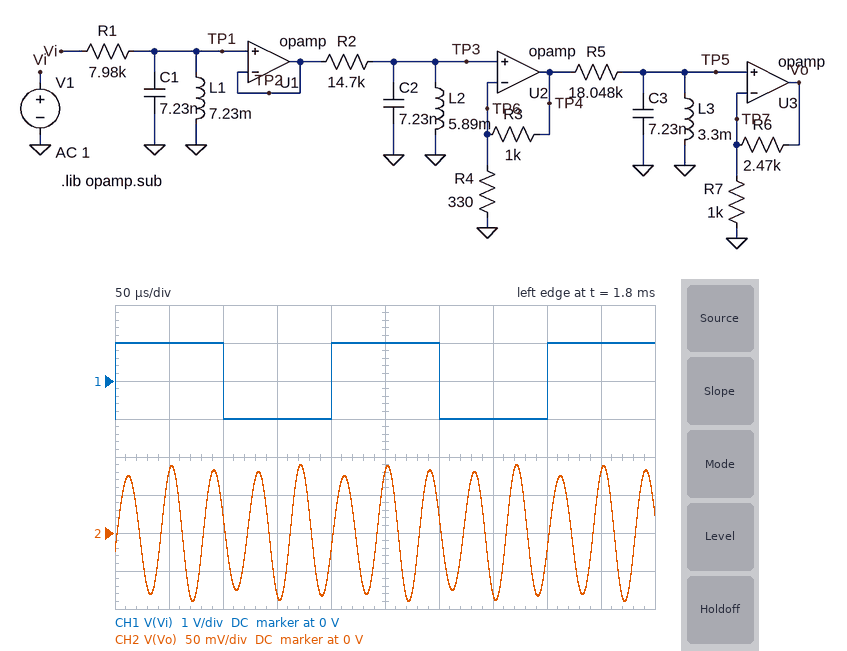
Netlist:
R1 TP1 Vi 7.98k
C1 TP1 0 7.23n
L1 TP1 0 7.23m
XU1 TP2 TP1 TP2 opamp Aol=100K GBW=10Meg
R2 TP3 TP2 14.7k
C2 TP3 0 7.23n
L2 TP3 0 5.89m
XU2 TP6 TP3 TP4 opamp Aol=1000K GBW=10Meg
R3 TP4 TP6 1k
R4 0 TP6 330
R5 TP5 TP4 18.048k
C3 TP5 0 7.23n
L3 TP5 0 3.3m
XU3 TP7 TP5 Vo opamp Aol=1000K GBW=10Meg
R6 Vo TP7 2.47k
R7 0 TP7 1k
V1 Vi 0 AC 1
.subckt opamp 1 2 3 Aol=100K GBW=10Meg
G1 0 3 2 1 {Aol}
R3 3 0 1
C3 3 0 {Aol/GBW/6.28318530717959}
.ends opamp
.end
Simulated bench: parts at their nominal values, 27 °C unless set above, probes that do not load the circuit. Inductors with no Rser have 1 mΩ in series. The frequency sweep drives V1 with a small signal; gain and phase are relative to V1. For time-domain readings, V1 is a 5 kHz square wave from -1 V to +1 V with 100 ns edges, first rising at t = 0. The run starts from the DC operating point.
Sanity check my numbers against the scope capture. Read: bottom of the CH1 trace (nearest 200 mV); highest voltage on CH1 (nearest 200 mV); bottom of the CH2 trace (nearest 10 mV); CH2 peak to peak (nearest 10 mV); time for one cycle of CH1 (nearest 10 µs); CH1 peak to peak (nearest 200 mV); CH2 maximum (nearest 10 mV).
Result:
-1.0 V
1.0 V
-90 mV
180 mV
200 µs
2.0 V
90 mV
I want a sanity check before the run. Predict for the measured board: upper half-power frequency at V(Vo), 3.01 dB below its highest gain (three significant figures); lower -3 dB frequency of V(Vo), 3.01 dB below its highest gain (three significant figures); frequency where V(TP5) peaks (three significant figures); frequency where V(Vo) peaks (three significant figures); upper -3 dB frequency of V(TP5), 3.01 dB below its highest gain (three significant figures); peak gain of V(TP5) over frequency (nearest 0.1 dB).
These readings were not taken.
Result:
25.0 kHz
23.4 kHz
24.3 kHz
24.3 kHz
25.0 kHz
-17.4 dB
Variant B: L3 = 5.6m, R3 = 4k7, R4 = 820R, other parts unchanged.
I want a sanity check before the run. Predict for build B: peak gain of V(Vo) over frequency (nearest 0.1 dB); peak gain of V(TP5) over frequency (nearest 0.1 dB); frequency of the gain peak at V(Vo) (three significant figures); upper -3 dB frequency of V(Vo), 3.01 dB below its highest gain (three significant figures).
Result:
19.2 dB
8.4 dB
24.7 kHz
25.2 kHz
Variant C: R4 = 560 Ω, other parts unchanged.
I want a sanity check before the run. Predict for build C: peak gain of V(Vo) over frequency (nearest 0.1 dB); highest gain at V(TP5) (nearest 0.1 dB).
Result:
-9.8 dB
-20.6 dB
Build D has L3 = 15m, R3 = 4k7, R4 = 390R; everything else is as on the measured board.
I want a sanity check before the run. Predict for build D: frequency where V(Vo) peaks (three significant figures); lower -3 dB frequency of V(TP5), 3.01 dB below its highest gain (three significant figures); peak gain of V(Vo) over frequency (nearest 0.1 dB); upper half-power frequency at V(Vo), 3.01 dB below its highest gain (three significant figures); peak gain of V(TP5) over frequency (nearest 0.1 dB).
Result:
24.1 kHz
22.2 kHz
6.1 dB
24.8 kHz
-4.7 dB
